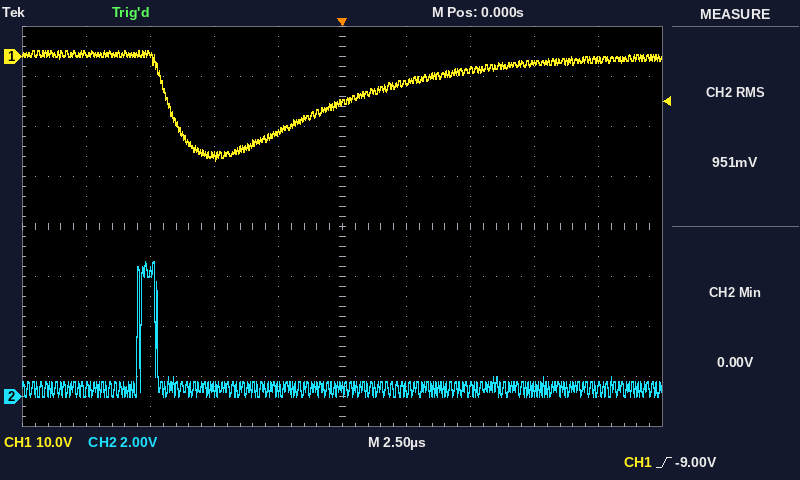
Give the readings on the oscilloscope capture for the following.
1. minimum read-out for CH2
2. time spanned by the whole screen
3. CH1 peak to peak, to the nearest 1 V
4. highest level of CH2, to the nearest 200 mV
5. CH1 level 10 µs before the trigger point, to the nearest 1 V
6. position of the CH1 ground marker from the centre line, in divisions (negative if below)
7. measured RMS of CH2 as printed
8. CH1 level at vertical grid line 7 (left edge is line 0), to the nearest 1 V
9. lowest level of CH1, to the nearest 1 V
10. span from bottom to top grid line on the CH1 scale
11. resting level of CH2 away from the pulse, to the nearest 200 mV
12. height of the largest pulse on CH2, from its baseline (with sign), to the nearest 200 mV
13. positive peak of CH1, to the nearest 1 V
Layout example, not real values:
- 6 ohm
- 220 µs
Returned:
- 0.00 V
- 25 µs
- 22 V
- 5.4 V
- 1 V
- +3.4 div
- 951 mV
- -3 V
- -21 V
- 80 V
- 400 mV
- +5.0 V
- 1 V
